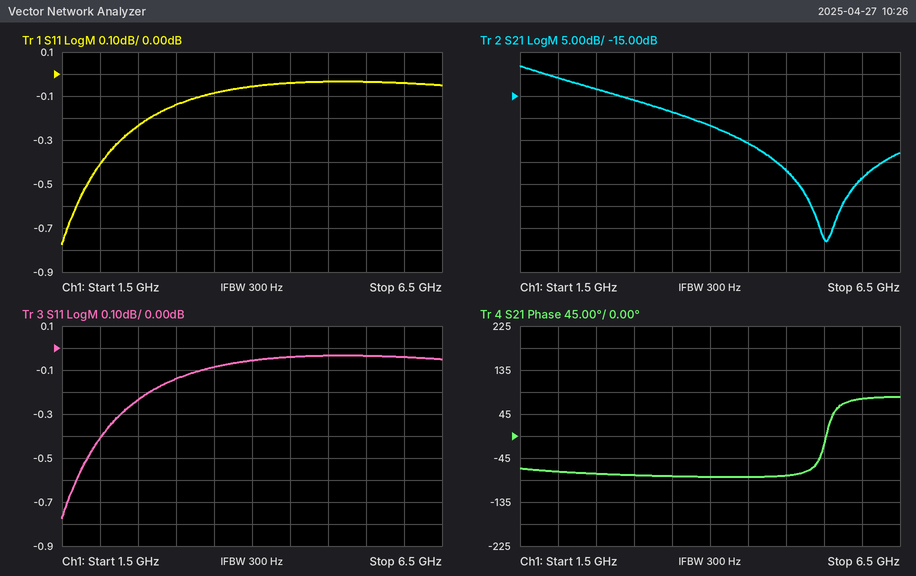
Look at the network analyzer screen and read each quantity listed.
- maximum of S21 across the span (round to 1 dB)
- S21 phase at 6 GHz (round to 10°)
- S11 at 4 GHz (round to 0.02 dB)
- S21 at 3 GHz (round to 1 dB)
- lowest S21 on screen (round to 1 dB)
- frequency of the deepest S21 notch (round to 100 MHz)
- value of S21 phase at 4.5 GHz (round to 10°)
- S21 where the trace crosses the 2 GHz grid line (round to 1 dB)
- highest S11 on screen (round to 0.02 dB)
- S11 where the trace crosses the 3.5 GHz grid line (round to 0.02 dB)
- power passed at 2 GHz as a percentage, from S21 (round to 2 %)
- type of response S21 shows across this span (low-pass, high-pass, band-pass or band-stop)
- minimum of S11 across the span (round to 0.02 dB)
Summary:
-8 dB
80°
-0.06 dB
-16 dB
-48 dB
5.5 GHz
-80°
-11 dB
-0.04 dB
-0.08 dB
8 %
low-pass
-0.78 dB
